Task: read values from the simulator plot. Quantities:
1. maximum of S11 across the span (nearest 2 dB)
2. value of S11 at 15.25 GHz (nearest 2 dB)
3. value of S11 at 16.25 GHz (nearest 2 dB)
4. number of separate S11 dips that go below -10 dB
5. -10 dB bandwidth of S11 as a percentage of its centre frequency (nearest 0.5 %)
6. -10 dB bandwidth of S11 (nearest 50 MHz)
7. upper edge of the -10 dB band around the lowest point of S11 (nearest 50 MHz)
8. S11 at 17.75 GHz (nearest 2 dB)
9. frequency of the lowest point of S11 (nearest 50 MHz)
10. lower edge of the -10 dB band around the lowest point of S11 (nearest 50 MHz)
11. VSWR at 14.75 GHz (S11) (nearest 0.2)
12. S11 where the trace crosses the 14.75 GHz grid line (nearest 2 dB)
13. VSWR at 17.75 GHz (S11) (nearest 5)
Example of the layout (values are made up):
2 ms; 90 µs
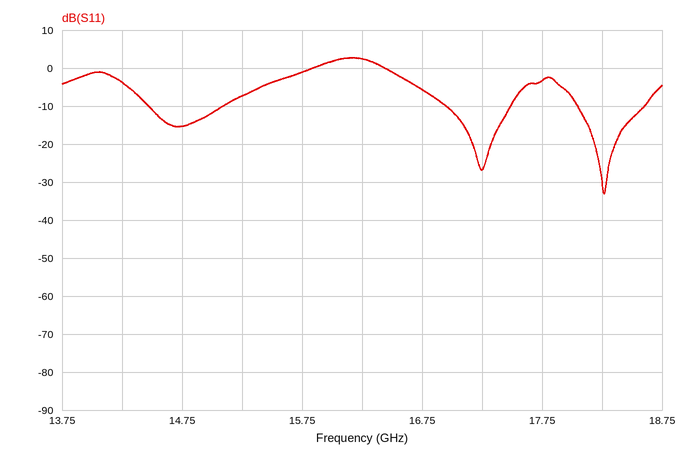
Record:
2 dB; -8 dB; 2 dB; 3; 3.0 %; 550 MHz; 18.60 GHz; -4 dB; 18.25 GHz; 18.05 GHz; 1.4; -16 dB; 5
